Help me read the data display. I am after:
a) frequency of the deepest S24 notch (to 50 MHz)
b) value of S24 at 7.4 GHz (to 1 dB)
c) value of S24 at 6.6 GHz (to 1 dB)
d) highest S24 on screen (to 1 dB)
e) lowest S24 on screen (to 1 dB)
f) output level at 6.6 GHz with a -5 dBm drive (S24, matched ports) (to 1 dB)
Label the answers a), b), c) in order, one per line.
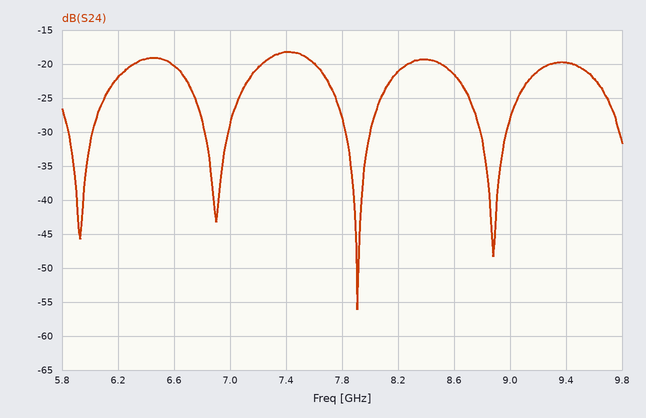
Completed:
a) 7.90 GHz
b) -18 dB
c) -20 dB
d) -18 dB
e) -56 dB
f) -25 dBm
